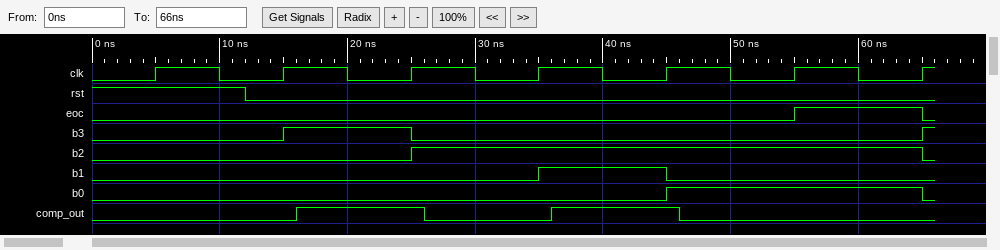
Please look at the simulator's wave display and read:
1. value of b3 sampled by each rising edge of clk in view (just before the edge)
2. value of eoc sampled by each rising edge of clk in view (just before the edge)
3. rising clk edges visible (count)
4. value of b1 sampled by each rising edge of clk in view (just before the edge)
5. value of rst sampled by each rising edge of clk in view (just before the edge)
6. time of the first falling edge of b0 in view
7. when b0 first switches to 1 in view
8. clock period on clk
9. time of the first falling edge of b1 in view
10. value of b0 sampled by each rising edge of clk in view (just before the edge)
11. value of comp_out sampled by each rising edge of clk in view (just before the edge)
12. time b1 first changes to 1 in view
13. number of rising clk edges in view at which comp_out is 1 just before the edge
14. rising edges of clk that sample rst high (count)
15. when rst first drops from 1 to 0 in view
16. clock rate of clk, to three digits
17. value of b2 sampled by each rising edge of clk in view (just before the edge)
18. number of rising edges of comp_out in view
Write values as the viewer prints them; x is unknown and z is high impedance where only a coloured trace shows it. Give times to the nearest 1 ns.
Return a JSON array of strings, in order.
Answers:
["0 0 1 0 0 0 0", "0 0 0 0 0 0 1", "7", "0 0 0 0 1 0 0", "1 0 0 0 0 0 0", "65 ns", "45 ns", "10 ns", "45 ns", "0 0 0 0 0 1 1", "0 0 1 0 1 0 0", "35 ns", "2", "1", "12 ns", "100 MHz", "0 0 0 1 1 1 1", "2"]
